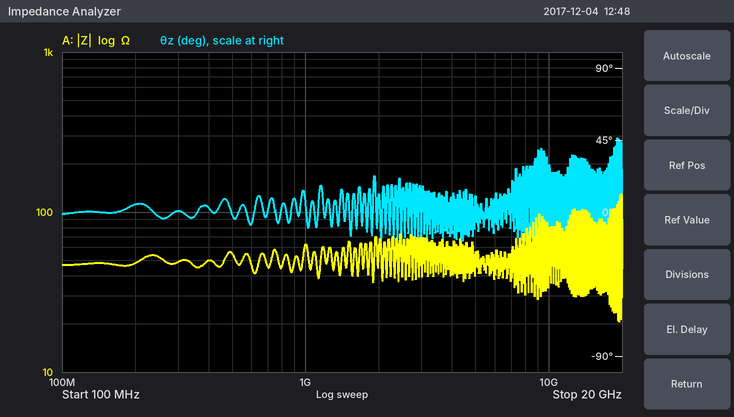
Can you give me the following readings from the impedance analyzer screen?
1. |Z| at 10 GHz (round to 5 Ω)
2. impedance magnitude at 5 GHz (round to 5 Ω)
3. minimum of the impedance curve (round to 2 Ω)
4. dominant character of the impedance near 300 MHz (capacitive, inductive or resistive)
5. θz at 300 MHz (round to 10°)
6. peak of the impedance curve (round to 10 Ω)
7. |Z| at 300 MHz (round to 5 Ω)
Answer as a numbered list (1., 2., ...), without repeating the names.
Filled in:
1. 55 Ω
2. 45 Ω
3. 20 Ω
4. resistive
5. 0°
6. 130 Ω
7. 50 Ω
